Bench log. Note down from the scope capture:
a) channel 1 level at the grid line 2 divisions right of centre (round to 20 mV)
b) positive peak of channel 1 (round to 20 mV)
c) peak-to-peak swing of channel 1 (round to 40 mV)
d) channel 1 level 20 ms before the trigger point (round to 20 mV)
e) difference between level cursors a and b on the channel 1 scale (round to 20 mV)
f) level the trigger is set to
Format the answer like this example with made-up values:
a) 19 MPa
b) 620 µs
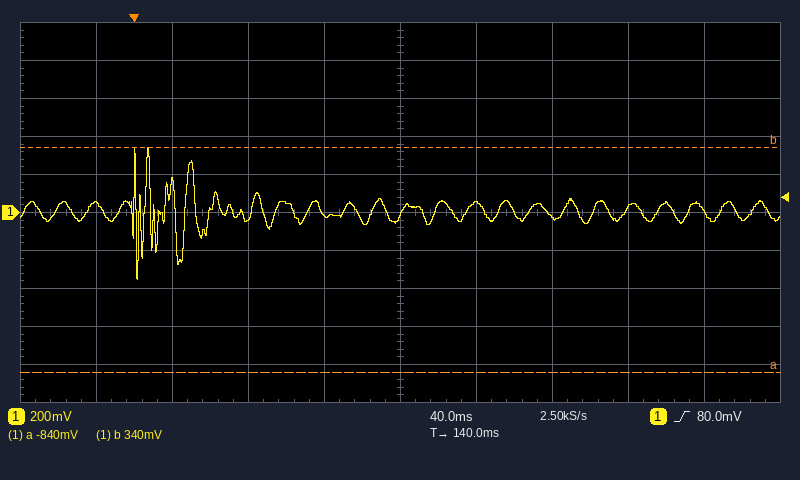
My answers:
a) -20 mV
b) 340 mV
c) 680 mV
d) 40 mV
e) 1.18 V
f) 80.0 mV
